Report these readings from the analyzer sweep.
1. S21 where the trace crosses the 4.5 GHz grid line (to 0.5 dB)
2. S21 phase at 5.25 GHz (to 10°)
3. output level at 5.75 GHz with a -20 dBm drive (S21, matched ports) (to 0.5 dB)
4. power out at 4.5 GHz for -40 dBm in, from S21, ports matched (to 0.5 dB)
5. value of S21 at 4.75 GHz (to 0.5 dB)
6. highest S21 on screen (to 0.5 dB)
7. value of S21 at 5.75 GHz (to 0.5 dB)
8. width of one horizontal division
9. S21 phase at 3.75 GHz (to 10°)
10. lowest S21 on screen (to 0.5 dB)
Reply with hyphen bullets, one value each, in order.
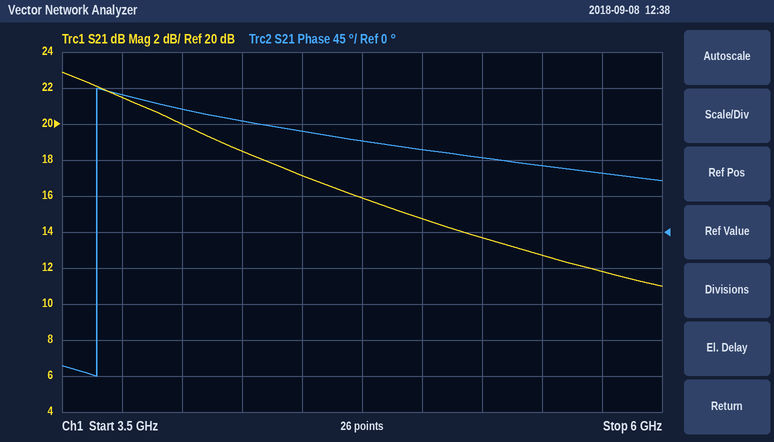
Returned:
- 17.0 dB
- 90°
- -8.0 dBm
- -23.0 dBm
- 16.0 dB
- 23.0 dB
- 12.0 dB
- 250 MHz
- 170°
- 11.0 dB
